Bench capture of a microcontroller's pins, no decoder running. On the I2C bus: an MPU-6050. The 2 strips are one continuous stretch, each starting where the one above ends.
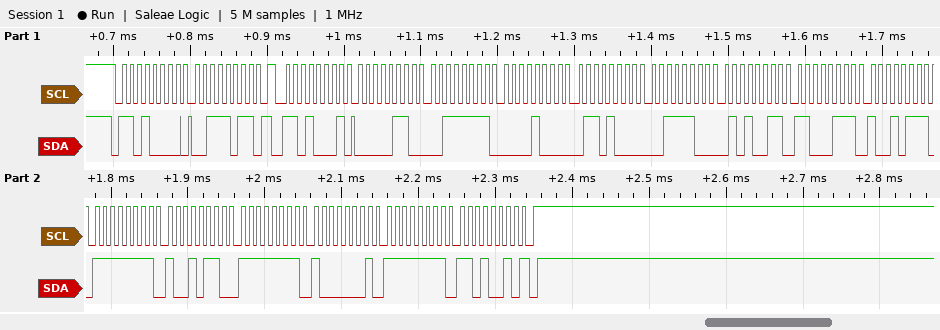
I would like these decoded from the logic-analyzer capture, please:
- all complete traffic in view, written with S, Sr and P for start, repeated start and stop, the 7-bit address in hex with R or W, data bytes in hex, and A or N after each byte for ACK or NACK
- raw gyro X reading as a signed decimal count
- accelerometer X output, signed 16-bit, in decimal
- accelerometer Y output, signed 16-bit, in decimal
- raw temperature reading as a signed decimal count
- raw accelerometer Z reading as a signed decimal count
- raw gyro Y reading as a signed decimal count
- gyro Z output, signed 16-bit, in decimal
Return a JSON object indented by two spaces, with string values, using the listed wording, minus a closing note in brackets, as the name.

{
  "all complete traffic in view, written with S, Sr and P for start, repeated start and stop, the 7-bit address in hex with R or W, data bytes in hex, and A or N after each byte for ACK or NACK": "S 68W A 3B A Sr 68R A 06 A 3F A 08 A 68 A 3C A 53 A C7 A 97 A FF A 96 A FF A 81 A FF A D2 N P",
  "raw gyro X reading as a signed decimal count": "-106",
  "accelerometer X output, signed 16-bit, in decimal": "1599",
  "accelerometer Y output, signed 16-bit, in decimal": "2152",
  "raw temperature reading as a signed decimal count": "-14441",
  "raw accelerometer Z reading as a signed decimal count": "15443",
  "raw gyro Y reading as a signed decimal count": "-127",
  "gyro Z output, signed 16-bit, in decimal": "-46"
}
